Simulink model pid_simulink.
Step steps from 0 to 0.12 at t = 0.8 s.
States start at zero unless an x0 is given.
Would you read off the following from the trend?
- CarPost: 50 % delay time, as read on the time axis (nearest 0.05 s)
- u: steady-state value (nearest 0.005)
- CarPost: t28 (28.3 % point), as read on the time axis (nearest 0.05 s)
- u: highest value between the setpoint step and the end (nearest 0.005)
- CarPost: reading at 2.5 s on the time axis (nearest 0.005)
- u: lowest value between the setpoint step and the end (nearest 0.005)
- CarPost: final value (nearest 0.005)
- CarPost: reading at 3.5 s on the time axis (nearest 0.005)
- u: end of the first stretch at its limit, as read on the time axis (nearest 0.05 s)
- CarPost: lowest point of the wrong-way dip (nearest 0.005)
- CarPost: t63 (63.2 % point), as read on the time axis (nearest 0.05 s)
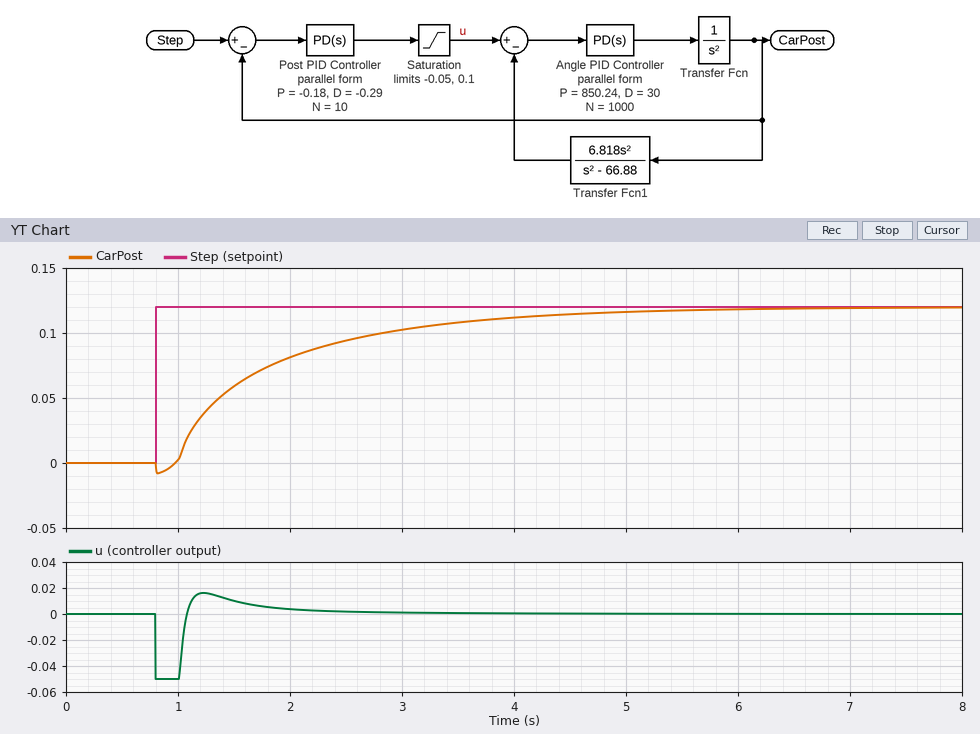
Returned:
1.50 s
0.000
1.20 s
0.015
0.095
-0.050
0.120
0.110
1.00 s
-0.010
1.85 s
